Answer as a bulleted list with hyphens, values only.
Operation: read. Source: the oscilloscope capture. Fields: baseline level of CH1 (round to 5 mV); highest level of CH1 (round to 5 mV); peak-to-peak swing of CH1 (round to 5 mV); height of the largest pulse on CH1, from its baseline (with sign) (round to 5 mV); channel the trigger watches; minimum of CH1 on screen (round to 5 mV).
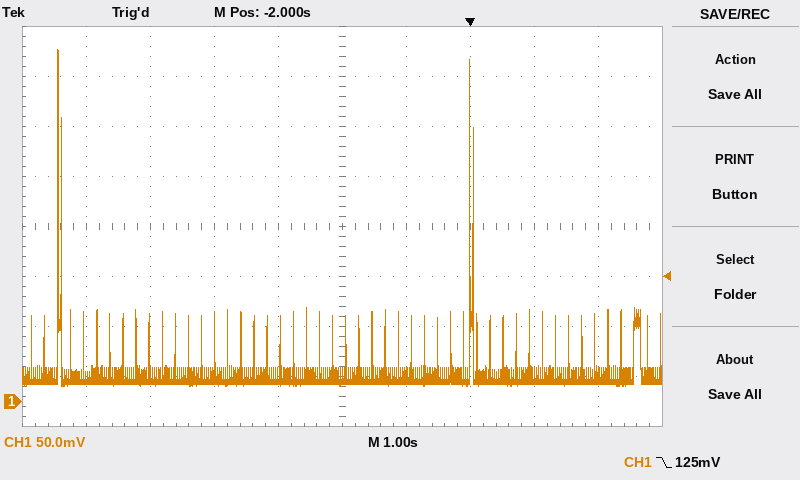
- 25 mV
- 350 mV
- 335 mV
- +325 mV
- CH1
- 15 mV
